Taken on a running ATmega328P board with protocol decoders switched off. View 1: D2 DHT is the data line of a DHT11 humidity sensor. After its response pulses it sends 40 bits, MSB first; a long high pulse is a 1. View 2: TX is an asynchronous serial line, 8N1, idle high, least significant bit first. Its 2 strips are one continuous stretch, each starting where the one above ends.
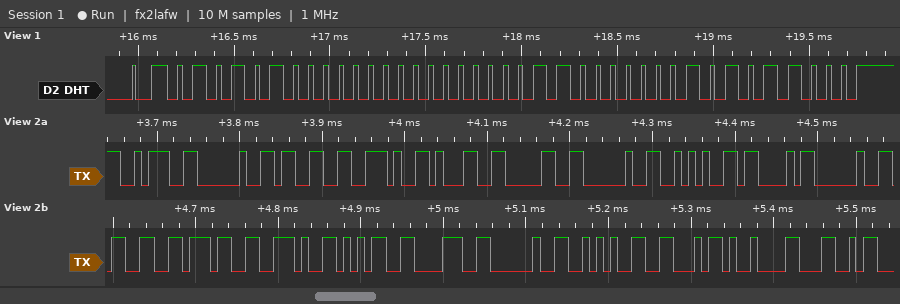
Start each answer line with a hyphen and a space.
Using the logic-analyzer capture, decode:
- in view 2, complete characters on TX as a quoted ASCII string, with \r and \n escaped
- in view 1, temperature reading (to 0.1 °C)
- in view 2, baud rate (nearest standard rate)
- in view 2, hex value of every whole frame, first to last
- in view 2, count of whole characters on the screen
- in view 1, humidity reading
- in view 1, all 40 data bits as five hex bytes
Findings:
- ": 3.10 *C 37.58 *F\tL"
- 3.1 °C
- 115200 baud
- 3A 20 33 2E 31 30 20 2A 43 20 33 37 2E 35 38 20 2A 46 09 4C
- 20
- 84 %
- 54 00 03 01 58
